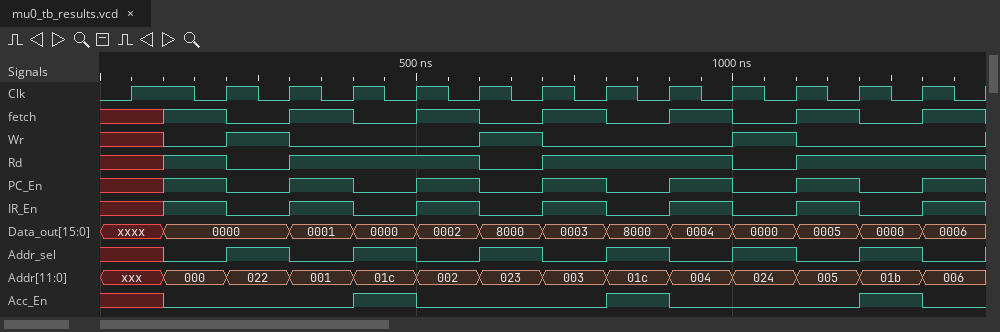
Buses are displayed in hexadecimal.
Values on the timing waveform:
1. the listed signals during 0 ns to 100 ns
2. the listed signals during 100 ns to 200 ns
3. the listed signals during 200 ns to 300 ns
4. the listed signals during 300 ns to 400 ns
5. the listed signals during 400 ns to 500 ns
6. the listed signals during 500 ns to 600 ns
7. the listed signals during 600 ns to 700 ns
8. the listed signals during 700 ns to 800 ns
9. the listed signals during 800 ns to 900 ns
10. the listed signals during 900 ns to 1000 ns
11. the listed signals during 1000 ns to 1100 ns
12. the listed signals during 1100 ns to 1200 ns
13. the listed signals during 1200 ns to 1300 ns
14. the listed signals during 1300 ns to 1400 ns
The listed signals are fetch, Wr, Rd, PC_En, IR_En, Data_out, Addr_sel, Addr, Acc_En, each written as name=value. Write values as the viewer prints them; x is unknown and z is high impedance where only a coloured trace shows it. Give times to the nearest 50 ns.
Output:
fetch=x, Wr=x, Rd=x, PC_En=x, IR_En=x, Data_out=xxxx, Addr_sel=x, Addr=xxx, Acc_En=x
fetch=1, Wr=0, Rd=1, PC_En=1, IR_En=1, Data_out=0000, Addr_sel=0, Addr=000, Acc_En=0
fetch=0, Wr=1, Rd=0, PC_En=0, IR_En=0, Data_out=0000, Addr_sel=1, Addr=022, Acc_En=0
fetch=1, Wr=0, Rd=1, PC_En=1, IR_En=1, Data_out=0001, Addr_sel=0, Addr=001, Acc_En=0
fetch=0, Wr=0, Rd=1, PC_En=0, IR_En=0, Data_out=0000, Addr_sel=1, Addr=01c, Acc_En=1
fetch=1, Wr=0, Rd=1, PC_En=1, IR_En=1, Data_out=0002, Addr_sel=0, Addr=002, Acc_En=0
fetch=0, Wr=1, Rd=0, PC_En=0, IR_En=0, Data_out=8000, Addr_sel=1, Addr=023, Acc_En=0
fetch=1, Wr=0, Rd=1, PC_En=1, IR_En=1, Data_out=0003, Addr_sel=0, Addr=003, Acc_En=0
fetch=0, Wr=0, Rd=1, PC_En=0, IR_En=0, Data_out=8000, Addr_sel=1, Addr=01c, Acc_En=1
fetch=1, Wr=0, Rd=1, PC_En=1, IR_En=1, Data_out=0004, Addr_sel=0, Addr=004, Acc_En=0
fetch=0, Wr=1, Rd=0, PC_En=0, IR_En=0, Data_out=0000, Addr_sel=1, Addr=024, Acc_En=0
fetch=1, Wr=0, Rd=1, PC_En=1, IR_En=1, Data_out=0005, Addr_sel=0, Addr=005, Acc_En=0
fetch=0, Wr=0, Rd=1, PC_En=0, IR_En=0, Data_out=0000, Addr_sel=1, Addr=01b, Acc_En=1
fetch=1, Wr=0, Rd=1, PC_En=1, IR_En=1, Data_out=0006, Addr_sel=0, Addr=006, Acc_En=0
